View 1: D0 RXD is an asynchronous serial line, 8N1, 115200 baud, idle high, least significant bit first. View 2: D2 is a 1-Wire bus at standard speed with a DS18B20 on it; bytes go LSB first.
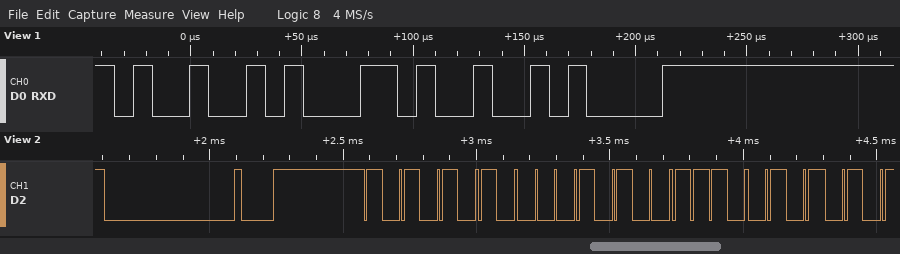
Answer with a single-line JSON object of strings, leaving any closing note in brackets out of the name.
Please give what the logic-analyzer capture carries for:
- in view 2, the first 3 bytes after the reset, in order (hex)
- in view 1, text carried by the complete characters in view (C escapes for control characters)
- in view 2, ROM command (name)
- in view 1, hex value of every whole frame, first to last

{"in view 2, the first 3 bytes after the reset, in order": "55 28 A7", "in view 1, text carried by the complete characters in view": "\"I,\\n\"", "in view 2, ROM command": "Match ROM", "in view 1, hex value of every whole frame, first to last": "49 2C 0A"}
